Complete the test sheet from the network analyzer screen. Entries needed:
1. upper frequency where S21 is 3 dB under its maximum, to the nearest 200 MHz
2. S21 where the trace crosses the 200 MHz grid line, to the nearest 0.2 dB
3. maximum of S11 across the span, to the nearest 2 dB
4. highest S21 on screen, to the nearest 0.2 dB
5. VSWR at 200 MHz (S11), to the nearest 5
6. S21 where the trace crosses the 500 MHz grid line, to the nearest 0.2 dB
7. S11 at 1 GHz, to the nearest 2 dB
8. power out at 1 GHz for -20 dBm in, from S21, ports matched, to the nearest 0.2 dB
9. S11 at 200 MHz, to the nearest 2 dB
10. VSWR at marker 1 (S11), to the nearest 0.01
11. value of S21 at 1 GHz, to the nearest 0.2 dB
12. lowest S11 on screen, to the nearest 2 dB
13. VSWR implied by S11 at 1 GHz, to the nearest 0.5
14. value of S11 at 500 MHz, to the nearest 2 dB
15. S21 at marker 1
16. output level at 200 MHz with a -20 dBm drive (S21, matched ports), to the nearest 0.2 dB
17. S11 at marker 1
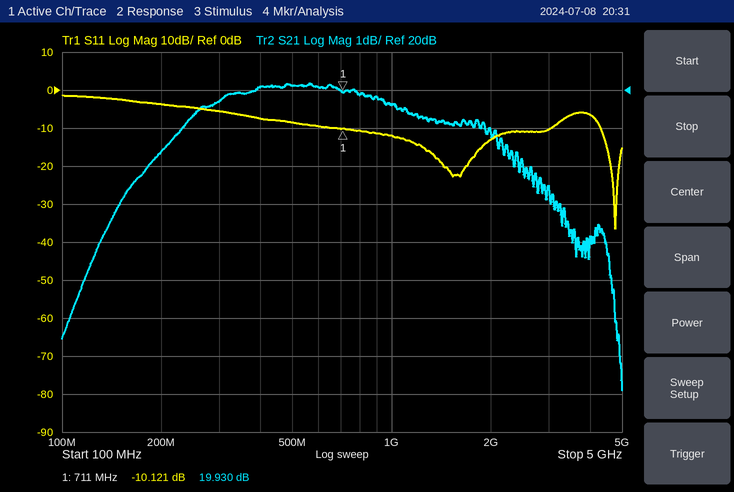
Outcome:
3.0 GHz
18.4 dB
-2 dB
20.2 dB
5
20.2 dB
-12 dB
-0.4 dBm
-4 dB
1.91
19.6 dB
-36 dB
1.5
-8 dB
19.930 dB
-1.6 dBm
-10.121 dB
